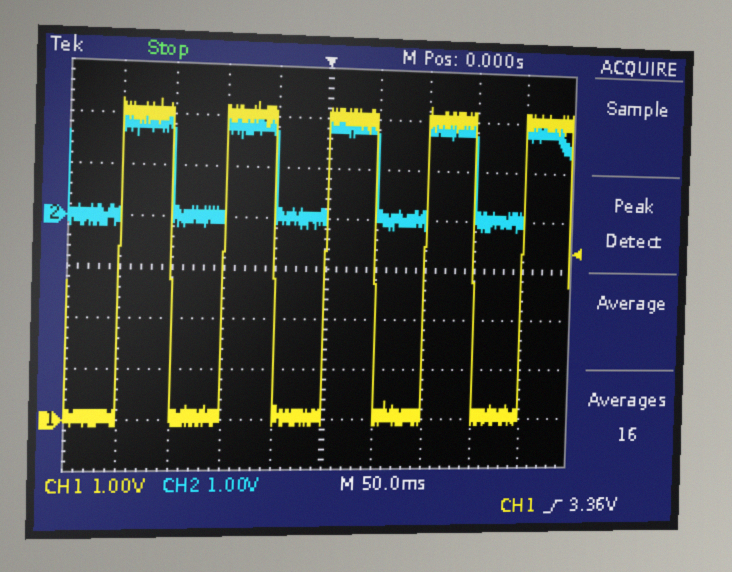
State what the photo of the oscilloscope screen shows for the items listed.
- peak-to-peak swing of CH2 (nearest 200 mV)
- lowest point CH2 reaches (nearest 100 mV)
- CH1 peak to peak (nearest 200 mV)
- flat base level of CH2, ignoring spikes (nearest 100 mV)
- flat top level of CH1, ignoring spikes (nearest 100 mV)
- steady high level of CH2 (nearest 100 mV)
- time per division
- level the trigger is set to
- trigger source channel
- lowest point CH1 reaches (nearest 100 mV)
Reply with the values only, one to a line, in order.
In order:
2.2 V
-200 mV
6.4 V
0.0 V
6.0 V
1.8 V
50 ms
3.36 V
CH1
-100 mV
